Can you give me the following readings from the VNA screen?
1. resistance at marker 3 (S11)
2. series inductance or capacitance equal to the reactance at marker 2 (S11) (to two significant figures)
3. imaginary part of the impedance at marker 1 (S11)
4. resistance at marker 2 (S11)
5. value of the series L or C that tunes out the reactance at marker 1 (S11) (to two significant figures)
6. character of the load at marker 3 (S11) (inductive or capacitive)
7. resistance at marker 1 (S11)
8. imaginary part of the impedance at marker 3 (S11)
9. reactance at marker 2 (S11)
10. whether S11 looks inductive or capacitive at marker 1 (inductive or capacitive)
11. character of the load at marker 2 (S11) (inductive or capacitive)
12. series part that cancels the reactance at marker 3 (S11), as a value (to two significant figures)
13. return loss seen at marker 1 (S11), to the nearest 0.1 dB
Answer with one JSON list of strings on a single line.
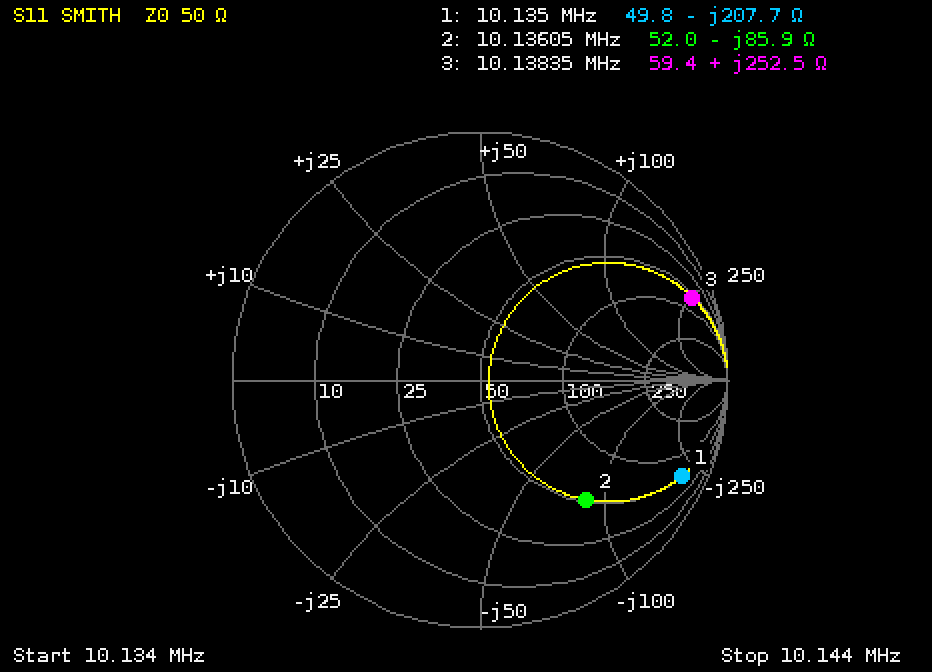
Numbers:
["59.4 Ω", "180 pF", "-207.7 Ω", "52.0 Ω", "3.3 µH", "inductive", "49.8 Ω", "+252.5 Ω", "-85.9 Ω", "capacitive", "capacitive", "62 pF", "0.9 dB"]
